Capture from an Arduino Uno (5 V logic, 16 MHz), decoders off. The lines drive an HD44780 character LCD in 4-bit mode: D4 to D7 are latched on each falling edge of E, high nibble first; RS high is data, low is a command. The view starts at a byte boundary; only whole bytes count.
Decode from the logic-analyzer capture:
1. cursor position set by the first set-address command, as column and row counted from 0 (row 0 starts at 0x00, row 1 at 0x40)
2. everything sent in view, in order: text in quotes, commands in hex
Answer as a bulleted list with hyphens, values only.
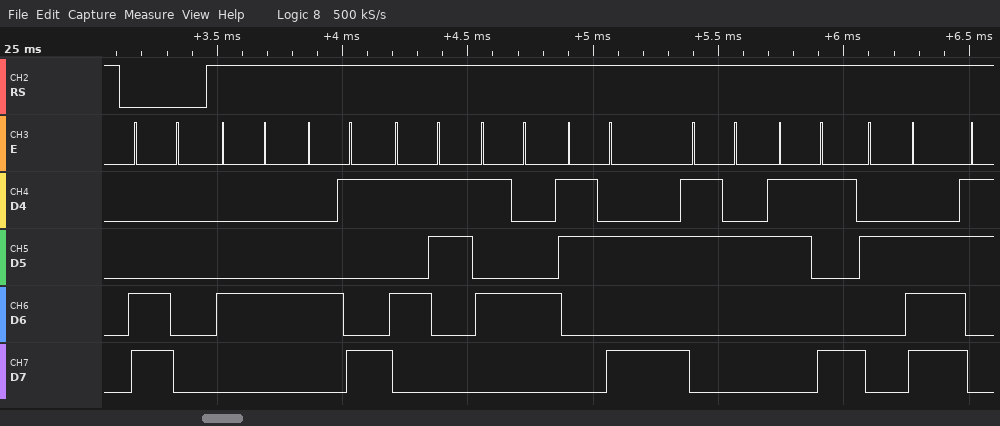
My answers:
- column 0, row 1
- 0xC0 "DIST:29."
